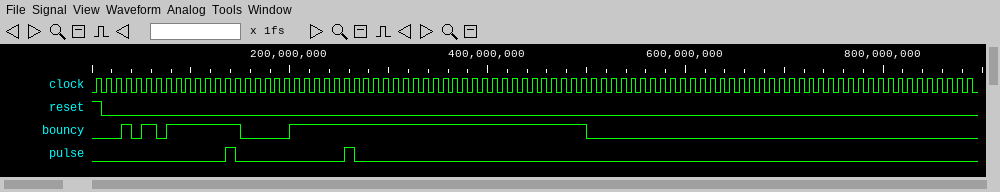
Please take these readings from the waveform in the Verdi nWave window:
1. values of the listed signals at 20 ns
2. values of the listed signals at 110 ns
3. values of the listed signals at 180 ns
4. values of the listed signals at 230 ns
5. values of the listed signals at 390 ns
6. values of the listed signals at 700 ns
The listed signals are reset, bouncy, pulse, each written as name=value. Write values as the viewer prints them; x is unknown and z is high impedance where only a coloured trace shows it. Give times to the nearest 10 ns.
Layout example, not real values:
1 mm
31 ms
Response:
reset=0, bouncy=0, pulse=0
reset=0, bouncy=1, pulse=0
reset=0, bouncy=0, pulse=0
reset=0, bouncy=1, pulse=0
reset=0, bouncy=1, pulse=0
reset=0, bouncy=0, pulse=0
